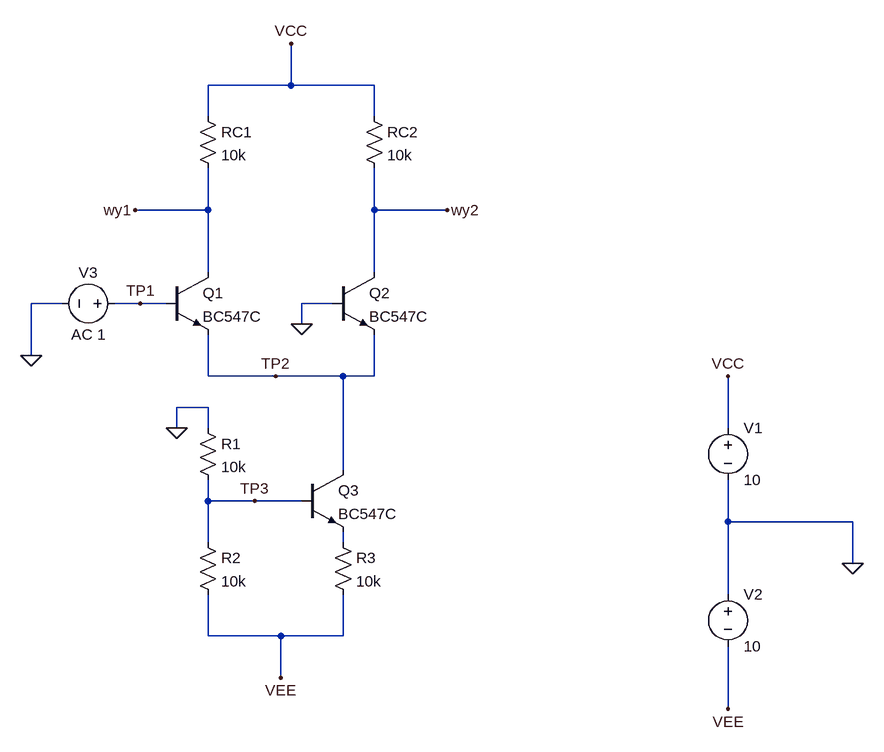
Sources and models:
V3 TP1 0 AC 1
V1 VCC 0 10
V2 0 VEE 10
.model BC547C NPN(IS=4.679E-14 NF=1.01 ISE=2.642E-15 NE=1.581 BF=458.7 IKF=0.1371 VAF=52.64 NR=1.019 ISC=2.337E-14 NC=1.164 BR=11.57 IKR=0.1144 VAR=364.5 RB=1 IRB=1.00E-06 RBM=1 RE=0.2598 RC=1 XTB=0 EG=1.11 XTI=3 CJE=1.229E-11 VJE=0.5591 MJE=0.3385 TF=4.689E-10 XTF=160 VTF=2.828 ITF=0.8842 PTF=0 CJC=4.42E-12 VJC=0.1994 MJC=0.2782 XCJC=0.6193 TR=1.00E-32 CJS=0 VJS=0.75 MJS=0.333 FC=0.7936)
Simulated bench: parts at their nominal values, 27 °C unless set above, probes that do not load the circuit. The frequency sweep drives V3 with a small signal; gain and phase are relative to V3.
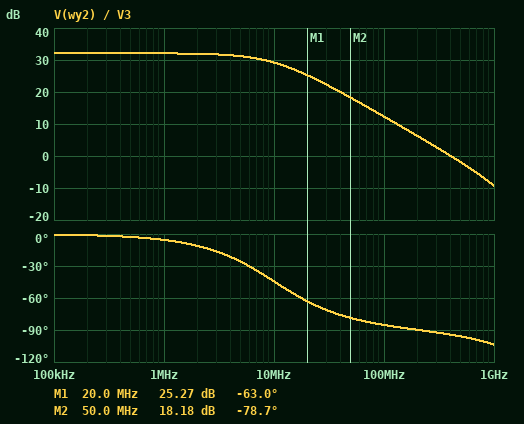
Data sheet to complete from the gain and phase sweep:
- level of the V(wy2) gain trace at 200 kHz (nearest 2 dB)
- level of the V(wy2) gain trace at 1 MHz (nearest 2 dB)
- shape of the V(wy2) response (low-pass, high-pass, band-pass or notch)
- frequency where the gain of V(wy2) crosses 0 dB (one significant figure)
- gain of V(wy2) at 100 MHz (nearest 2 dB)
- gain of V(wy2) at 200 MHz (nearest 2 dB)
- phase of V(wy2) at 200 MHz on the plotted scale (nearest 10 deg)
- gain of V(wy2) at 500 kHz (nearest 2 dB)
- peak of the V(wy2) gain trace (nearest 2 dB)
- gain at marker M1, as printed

32 dB
32 dB
low-pass
400 MHz
12 dB
6 dB
-90 deg
32 dB
32 dB
25.27 dB
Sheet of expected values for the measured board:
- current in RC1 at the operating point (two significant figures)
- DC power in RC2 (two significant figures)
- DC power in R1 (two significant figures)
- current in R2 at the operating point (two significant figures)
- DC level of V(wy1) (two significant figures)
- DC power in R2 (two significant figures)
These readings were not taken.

220 µA
480 µW
2.5 mW
500 µA
7.8 V
2.5 mW
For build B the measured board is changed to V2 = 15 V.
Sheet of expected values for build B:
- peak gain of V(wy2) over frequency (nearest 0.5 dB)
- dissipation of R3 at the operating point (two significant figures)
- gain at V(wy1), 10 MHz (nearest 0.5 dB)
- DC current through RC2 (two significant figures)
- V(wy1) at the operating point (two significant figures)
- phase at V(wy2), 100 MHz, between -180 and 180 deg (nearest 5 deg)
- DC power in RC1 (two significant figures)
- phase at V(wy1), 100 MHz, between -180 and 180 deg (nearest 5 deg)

36.0 dB
4.7 mW
33.0 dB
340 µA
6.6 V
-85 deg
1.2 mW
85 deg
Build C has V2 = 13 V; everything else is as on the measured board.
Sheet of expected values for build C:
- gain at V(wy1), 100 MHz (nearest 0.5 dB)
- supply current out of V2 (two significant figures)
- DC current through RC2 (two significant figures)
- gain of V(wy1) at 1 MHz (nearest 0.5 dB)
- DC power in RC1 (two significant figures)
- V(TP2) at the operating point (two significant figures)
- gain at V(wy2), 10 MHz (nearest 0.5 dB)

15.0 dB
1.2 mA
290 µA
34.5 dB
860 µW
-590 mV
31.5 dB
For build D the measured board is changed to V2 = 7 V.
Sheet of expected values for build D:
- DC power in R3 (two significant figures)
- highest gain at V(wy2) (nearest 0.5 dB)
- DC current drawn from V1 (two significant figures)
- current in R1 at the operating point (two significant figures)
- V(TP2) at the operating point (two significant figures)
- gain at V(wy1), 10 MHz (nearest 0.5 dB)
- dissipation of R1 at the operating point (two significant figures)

850 µW
28.5 dB
290 µA
350 µA
-570 mV
26.0 dB
1.2 mW
